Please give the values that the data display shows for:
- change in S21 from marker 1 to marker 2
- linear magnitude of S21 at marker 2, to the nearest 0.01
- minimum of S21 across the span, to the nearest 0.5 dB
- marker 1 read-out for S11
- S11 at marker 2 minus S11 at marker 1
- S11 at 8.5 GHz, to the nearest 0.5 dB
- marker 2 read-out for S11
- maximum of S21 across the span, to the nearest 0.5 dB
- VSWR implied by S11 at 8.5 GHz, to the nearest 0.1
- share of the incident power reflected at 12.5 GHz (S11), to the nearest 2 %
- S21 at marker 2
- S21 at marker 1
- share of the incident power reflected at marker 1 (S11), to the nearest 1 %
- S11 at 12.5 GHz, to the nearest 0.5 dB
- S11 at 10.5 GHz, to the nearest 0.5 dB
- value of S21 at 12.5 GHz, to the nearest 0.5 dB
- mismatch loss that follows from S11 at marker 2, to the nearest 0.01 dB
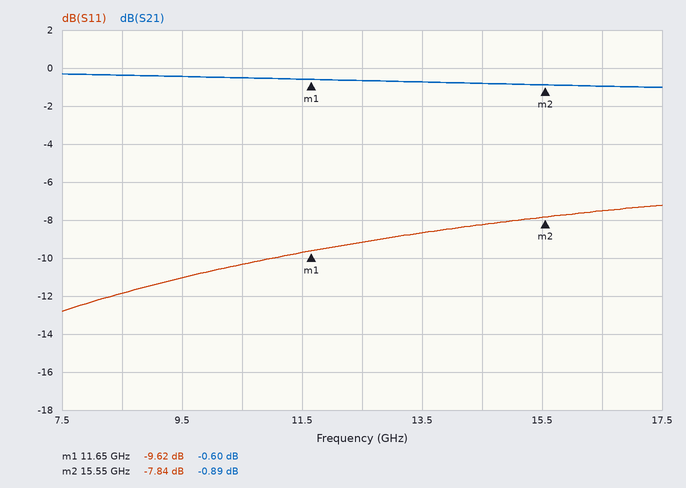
-0.29 dB
0.90
-1.0 dB
-9.62 dB
1.78 dB
-12.0 dB
-7.84 dB
-0.5 dB
1.7
12 %
-0.89 dB
-0.60 dB
11 %
-9.0 dB
-10.5 dB
-0.5 dB
0.78 dB
